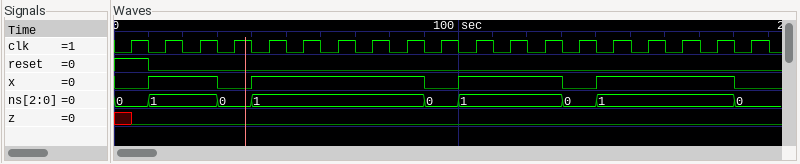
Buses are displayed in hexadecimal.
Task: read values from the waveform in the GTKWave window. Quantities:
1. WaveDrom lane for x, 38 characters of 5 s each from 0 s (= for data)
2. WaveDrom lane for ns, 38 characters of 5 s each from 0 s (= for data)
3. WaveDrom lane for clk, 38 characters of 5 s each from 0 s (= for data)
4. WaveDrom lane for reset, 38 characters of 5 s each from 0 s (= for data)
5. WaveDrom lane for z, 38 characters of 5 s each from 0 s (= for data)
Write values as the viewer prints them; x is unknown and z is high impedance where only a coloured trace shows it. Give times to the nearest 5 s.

{name: 'x', wave: '0.1...0.1.........0.1.....0.1.......0.'}
{name: 'ns', wave: '=.=...=.=.........=.=.....=.=.......=.', data: '0 1 0 1 0 1 0 1 0'}
{name: 'clk', wave: '01010101010101010101010101010101010101'}
{name: 'reset', wave: '1.0...................................'}
{name: 'z', wave: 'x0....................................'}
